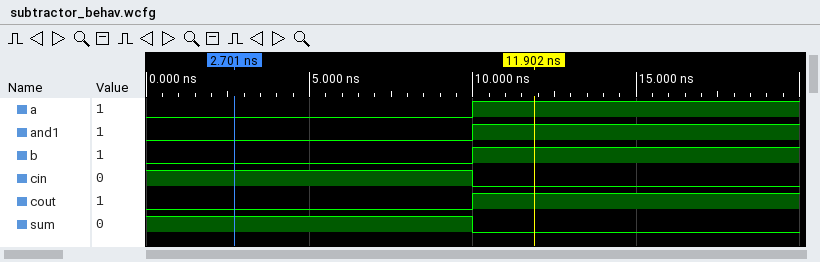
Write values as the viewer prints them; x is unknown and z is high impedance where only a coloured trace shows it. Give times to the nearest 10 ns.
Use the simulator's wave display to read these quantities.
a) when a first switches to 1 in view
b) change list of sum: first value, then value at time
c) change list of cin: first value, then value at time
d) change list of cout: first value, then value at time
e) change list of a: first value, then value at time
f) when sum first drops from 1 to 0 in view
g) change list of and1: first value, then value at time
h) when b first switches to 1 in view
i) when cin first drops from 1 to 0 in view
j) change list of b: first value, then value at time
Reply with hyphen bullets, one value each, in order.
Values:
- 10 ns
- 1, 0 at 10 ns
- 1, 0 at 10 ns
- 0, 1 at 10 ns
- 0, 1 at 10 ns
- 10 ns
- 0, 1 at 10 ns
- 10 ns
- 10 ns
- 0, 1 at 10 ns
